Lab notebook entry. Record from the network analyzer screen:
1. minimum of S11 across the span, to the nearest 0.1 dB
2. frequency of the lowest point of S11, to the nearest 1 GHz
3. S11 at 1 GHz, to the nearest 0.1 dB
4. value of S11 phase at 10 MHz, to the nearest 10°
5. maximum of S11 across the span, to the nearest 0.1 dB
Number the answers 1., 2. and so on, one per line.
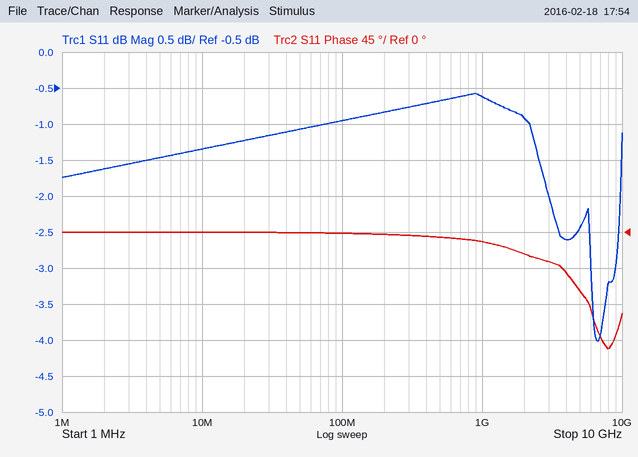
1. -4.0 dB
2. 7 GHz
3. -0.6 dB
4. 0°
5. -0.6 dB
